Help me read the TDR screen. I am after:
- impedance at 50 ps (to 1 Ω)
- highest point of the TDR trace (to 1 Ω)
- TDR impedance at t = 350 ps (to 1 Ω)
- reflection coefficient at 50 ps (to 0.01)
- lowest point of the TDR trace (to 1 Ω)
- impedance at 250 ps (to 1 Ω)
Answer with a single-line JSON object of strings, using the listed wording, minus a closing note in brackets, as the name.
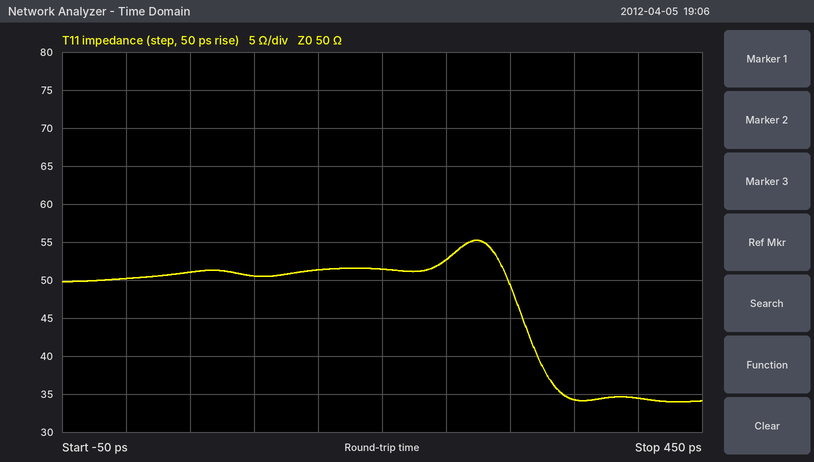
{"impedance at 50 ps": "51 Ω", "highest point of the TDR trace": "55 Ω", "TDR impedance at t = 350 ps": "34 Ω", "reflection coefficient at 50 ps": "+0.01", "lowest point of the TDR trace": "34 Ω", "impedance at 250 ps": "53 Ω"}
